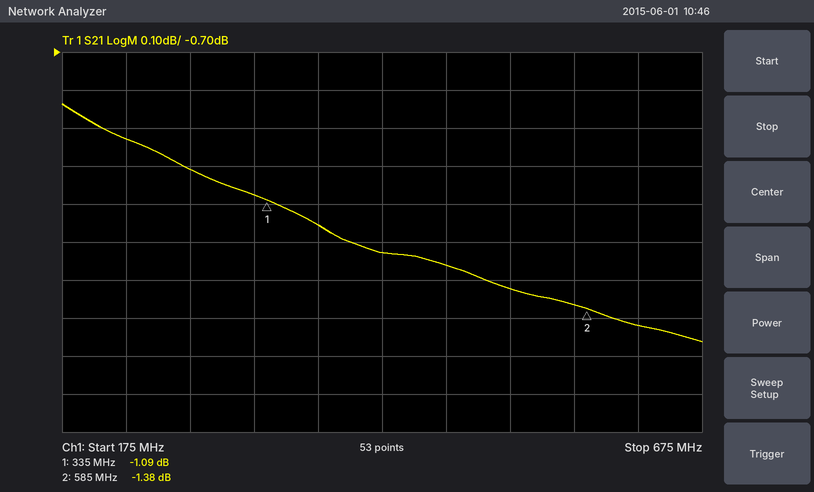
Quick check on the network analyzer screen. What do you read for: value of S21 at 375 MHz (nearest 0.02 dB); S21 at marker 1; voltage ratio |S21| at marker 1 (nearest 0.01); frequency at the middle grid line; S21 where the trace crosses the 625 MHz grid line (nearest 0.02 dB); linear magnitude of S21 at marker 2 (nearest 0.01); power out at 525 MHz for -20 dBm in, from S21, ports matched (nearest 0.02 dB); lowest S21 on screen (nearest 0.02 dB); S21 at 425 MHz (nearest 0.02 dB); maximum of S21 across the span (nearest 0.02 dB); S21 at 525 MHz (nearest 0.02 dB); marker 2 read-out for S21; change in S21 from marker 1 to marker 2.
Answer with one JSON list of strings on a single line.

["-1.16 dB", "-1.09 dB", "0.88", "425 MHz", "-1.42 dB", "0.85", "-21.32 dBm", "-1.46 dB", "-1.22 dB", "-0.84 dB", "-1.32 dB", "-1.38 dB", "-0.29 dB"]
